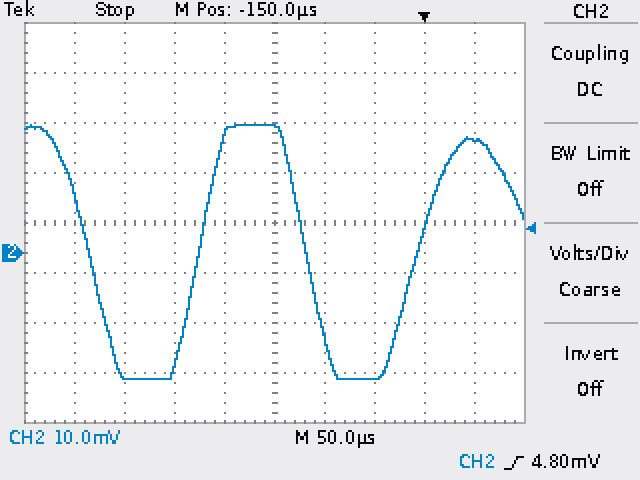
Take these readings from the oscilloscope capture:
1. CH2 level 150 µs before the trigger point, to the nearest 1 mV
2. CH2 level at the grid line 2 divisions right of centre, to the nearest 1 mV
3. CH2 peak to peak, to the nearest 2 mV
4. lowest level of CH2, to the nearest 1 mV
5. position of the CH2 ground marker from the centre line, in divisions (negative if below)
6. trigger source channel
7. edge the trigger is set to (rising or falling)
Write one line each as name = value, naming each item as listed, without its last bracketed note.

CH2 level 150 µs before the trigger point, to the nearest 1 mV = 25 mV
CH2 level at the grid line 2 divisions right of centre, to the nearest 1 mV = -25 mV
CH2 peak to peak, to the nearest 2 mV = 50 mV
lowest level of CH2, to the nearest 1 mV = -25 mV
position of the CH2 ground marker from the centre line, in divisions = -0.6 div
trigger source channel = CH2
edge the trigger is set to = rising
